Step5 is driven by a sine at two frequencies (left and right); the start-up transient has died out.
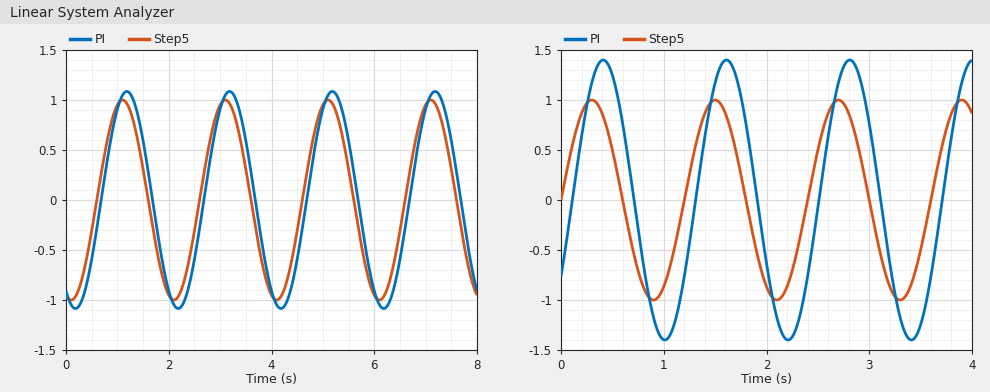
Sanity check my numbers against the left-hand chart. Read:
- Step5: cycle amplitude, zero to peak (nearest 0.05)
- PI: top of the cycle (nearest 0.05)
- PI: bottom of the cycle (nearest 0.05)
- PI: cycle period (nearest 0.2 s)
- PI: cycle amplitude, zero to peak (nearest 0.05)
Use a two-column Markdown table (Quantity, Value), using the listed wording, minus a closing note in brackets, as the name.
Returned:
| Quantity | Value |
|---|---|
| Step5: cycle amplitude, zero to peak | 1.00 |
| PI: top of the cycle | 1.10 |
| PI: bottom of the cycle | -1.10 |
| PI: cycle period | 2.0 s |
| PI: cycle amplitude, zero to peak | 1.10 |
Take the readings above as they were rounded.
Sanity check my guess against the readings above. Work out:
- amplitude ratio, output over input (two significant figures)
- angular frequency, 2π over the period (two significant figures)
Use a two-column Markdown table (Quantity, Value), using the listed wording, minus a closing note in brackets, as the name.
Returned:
| Quantity | Value |
|---|---|
| amplitude ratio, output over input | 1.1 |
| angular frequency, 2π over the period | 3.1 rad/s |
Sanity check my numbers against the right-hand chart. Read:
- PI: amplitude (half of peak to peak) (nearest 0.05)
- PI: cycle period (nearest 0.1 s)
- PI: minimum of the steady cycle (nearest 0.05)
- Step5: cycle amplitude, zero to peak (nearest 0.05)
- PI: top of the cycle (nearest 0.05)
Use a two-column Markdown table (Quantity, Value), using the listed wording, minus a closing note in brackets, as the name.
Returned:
| Quantity | Value |
|---|---|
| PI: amplitude (half of peak to peak) | 1.40 |
| PI: cycle period | 1.2 s |
| PI: minimum of the steady cycle | -1.40 |
| Step5: cycle amplitude, zero to peak | 1.00 |
| PI: top of the cycle | 1.40 |
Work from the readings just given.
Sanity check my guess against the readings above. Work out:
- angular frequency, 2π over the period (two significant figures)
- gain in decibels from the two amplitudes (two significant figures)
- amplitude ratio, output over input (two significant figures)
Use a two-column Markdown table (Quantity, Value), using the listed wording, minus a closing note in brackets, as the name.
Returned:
| Quantity | Value |
|---|---|
| angular frequency, 2π over the period | 5.2 rad/s |
| gain in decibels from the two amplitudes | 2.9 dB |
| amplitude ratio, output over input | 1.4 |
